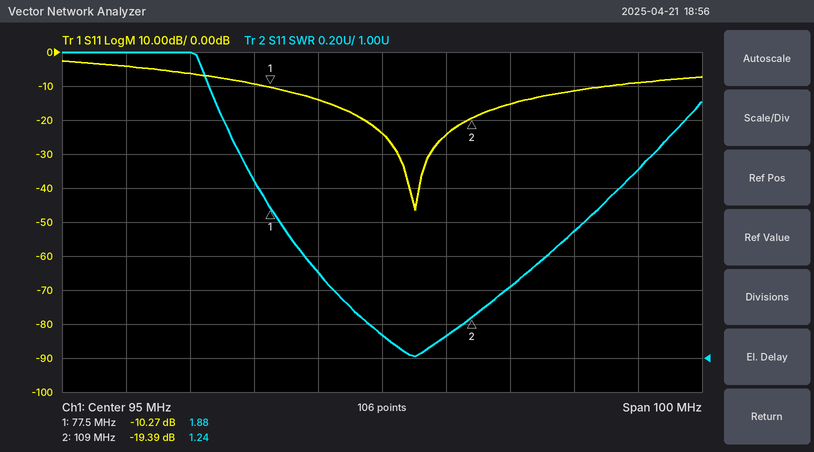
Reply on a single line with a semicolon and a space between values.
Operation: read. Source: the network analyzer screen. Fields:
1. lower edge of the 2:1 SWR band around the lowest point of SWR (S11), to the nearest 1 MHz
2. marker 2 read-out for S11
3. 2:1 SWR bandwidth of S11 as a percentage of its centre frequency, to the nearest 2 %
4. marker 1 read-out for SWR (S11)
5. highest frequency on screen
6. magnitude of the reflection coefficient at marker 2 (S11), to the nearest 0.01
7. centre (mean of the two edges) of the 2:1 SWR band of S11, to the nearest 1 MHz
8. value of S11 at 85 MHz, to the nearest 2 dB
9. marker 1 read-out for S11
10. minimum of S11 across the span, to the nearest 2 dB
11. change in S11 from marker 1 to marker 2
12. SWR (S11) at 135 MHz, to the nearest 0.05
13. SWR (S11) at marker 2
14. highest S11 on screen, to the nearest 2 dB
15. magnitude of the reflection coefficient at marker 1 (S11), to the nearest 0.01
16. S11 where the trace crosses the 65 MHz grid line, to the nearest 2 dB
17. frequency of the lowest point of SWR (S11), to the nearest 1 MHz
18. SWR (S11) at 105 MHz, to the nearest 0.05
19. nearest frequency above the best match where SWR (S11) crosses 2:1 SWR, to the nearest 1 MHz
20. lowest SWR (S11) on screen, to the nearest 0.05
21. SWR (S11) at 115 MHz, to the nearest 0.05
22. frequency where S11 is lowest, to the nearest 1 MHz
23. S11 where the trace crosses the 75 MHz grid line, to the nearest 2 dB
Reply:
76 MHz; -19.39 dB; 54 %; 1.88; 145 MHz; 0.11; 104 MHz; -14 dB; -10.27 dB; -46 dB; -9.12 dB; 2.10; 1.24; -2 dB; 0.31; -6 dB; 100 MHz; 1.15; 132 MHz; 1.00; 1.40; 100 MHz; -10 dB
